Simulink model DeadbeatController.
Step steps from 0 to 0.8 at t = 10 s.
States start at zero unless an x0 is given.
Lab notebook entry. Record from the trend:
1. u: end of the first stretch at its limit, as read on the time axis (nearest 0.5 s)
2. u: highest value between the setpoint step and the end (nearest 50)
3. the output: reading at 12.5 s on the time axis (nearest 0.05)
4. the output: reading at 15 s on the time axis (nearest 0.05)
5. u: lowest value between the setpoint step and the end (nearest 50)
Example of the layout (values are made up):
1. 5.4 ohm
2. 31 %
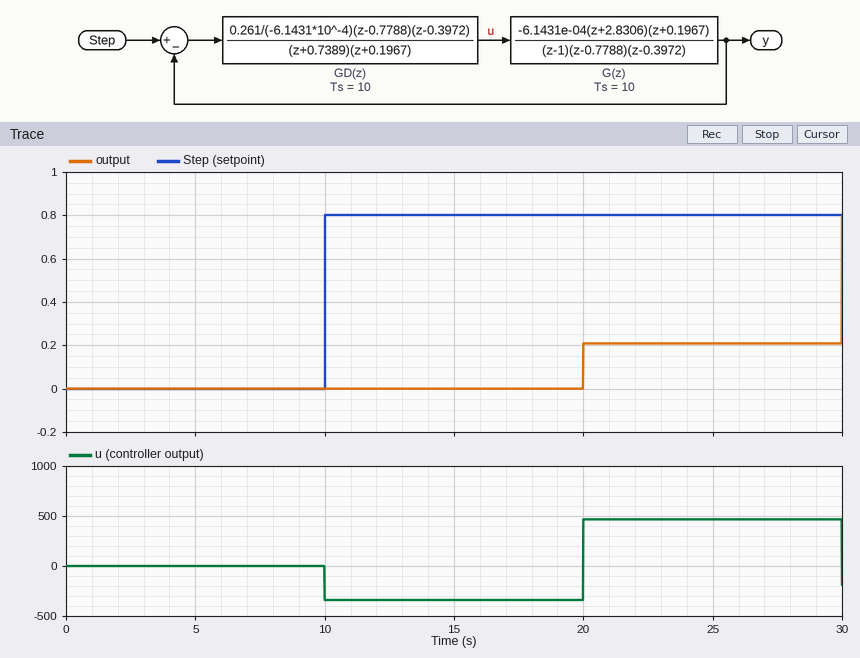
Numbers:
1. 20.0 s
2. 450
3. 0.00
4. 0.00
5. -350
